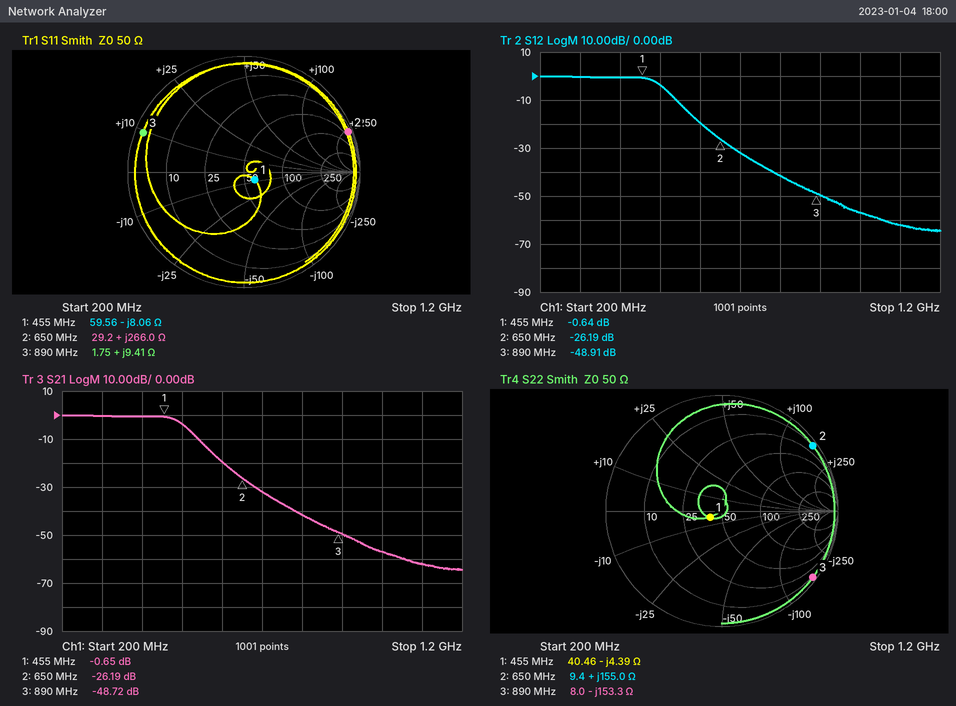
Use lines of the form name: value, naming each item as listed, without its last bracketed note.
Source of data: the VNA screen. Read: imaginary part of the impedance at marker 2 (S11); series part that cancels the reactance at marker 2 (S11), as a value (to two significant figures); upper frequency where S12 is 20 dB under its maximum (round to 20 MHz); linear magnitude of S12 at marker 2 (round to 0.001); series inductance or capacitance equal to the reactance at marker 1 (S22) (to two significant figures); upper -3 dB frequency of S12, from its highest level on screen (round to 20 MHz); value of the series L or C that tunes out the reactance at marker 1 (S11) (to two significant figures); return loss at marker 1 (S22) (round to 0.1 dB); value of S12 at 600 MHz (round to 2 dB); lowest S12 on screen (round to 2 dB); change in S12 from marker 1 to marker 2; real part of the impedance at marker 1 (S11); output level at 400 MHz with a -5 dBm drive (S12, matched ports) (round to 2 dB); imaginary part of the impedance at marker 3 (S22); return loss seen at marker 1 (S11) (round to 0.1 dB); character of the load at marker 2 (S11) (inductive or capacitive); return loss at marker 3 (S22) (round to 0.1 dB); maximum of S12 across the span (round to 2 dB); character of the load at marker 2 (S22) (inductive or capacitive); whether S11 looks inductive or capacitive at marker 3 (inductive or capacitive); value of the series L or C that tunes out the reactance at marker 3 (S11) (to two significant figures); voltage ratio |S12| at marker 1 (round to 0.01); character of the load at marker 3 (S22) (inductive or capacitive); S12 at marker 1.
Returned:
imaginary part of the impedance at marker 2: +266.0 Ω
series part that cancels the reactance at marker 2 (S11), as a value: 920 fF
upper frequency where S12 is 20 dB under its maximum: 600 MHz
linear magnitude of S12 at marker 2: 0.049
series inductance or capacitance equal to the reactance at marker 1 (S22): 80 pF
upper -3 dB frequency of S12, from its highest level on screen: 500 MHz
value of the series L or C that tunes out the reactance at marker 1 (S11): 2.8 nH
return loss at marker 1 (S22): 18.7 dB
value of S12 at 600 MHz: -20 dB
lowest S12 on screen: -64 dB
change in S12 from marker 1 to marker 2: -25.55 dB
real part of the impedance at marker 1: 59.56 Ω
output level at 400 MHz with a -5 dBm drive (S12, matched ports): -6 dBm
imaginary part of the impedance at marker 3: -153.3 Ω
return loss seen at marker 1 (S11): 18.9 dB
character of the load at marker 2 (S11): inductive
return loss at marker 3 (S22): 0.3 dB
maximum of S12 across the span: 0 dB
character of the load at marker 2 (S22): inductive
whether S11 looks inductive or capacitive at marker 3: inductive
value of the series L or C that tunes out the reactance at marker 3 (S11): 19 pF
voltage ratio |S12| at marker 1: 0.93
character of the load at marker 3 (S22): capacitive
S12 at marker 1: -0.64 dB
